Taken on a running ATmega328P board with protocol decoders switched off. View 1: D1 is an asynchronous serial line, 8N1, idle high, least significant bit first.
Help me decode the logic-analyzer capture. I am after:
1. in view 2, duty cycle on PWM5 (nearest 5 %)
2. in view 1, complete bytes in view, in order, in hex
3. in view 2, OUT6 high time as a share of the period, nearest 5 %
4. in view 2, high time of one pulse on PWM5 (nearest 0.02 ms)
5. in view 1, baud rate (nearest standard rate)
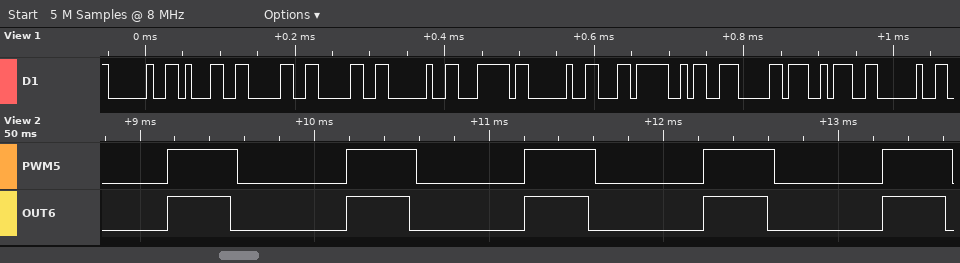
40 %
20 31 30 30 20 7C 20 EC 9A B0 3A 20
35 %
0.40 ms
115200 baud
